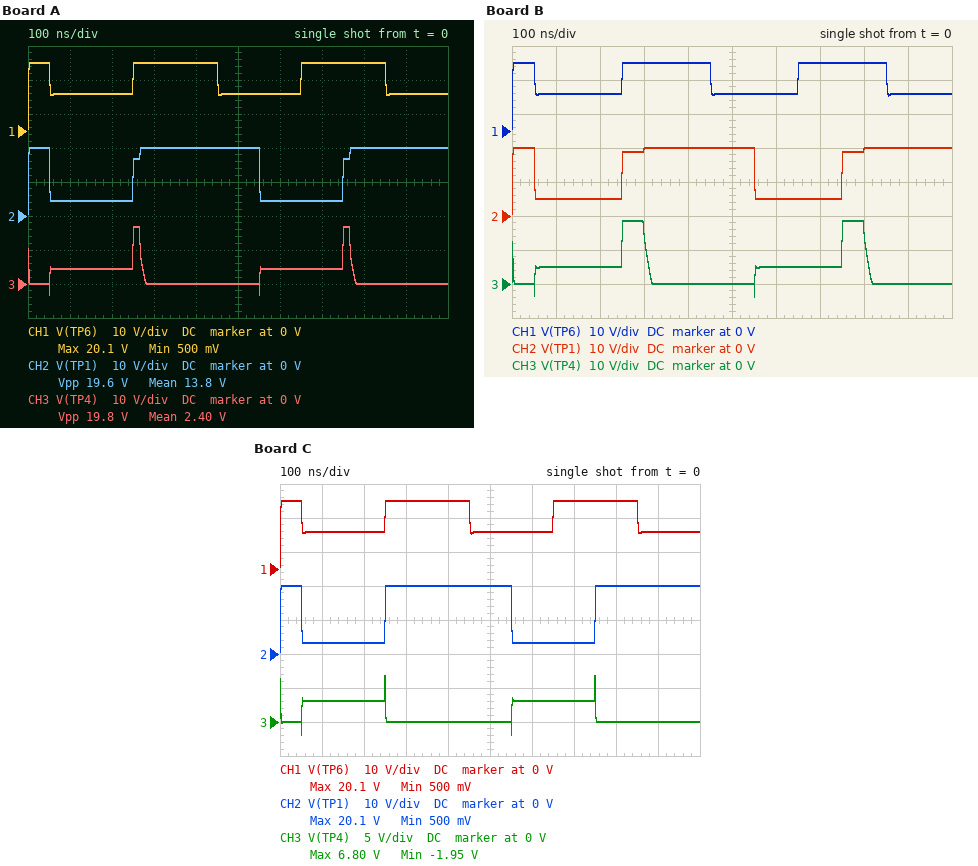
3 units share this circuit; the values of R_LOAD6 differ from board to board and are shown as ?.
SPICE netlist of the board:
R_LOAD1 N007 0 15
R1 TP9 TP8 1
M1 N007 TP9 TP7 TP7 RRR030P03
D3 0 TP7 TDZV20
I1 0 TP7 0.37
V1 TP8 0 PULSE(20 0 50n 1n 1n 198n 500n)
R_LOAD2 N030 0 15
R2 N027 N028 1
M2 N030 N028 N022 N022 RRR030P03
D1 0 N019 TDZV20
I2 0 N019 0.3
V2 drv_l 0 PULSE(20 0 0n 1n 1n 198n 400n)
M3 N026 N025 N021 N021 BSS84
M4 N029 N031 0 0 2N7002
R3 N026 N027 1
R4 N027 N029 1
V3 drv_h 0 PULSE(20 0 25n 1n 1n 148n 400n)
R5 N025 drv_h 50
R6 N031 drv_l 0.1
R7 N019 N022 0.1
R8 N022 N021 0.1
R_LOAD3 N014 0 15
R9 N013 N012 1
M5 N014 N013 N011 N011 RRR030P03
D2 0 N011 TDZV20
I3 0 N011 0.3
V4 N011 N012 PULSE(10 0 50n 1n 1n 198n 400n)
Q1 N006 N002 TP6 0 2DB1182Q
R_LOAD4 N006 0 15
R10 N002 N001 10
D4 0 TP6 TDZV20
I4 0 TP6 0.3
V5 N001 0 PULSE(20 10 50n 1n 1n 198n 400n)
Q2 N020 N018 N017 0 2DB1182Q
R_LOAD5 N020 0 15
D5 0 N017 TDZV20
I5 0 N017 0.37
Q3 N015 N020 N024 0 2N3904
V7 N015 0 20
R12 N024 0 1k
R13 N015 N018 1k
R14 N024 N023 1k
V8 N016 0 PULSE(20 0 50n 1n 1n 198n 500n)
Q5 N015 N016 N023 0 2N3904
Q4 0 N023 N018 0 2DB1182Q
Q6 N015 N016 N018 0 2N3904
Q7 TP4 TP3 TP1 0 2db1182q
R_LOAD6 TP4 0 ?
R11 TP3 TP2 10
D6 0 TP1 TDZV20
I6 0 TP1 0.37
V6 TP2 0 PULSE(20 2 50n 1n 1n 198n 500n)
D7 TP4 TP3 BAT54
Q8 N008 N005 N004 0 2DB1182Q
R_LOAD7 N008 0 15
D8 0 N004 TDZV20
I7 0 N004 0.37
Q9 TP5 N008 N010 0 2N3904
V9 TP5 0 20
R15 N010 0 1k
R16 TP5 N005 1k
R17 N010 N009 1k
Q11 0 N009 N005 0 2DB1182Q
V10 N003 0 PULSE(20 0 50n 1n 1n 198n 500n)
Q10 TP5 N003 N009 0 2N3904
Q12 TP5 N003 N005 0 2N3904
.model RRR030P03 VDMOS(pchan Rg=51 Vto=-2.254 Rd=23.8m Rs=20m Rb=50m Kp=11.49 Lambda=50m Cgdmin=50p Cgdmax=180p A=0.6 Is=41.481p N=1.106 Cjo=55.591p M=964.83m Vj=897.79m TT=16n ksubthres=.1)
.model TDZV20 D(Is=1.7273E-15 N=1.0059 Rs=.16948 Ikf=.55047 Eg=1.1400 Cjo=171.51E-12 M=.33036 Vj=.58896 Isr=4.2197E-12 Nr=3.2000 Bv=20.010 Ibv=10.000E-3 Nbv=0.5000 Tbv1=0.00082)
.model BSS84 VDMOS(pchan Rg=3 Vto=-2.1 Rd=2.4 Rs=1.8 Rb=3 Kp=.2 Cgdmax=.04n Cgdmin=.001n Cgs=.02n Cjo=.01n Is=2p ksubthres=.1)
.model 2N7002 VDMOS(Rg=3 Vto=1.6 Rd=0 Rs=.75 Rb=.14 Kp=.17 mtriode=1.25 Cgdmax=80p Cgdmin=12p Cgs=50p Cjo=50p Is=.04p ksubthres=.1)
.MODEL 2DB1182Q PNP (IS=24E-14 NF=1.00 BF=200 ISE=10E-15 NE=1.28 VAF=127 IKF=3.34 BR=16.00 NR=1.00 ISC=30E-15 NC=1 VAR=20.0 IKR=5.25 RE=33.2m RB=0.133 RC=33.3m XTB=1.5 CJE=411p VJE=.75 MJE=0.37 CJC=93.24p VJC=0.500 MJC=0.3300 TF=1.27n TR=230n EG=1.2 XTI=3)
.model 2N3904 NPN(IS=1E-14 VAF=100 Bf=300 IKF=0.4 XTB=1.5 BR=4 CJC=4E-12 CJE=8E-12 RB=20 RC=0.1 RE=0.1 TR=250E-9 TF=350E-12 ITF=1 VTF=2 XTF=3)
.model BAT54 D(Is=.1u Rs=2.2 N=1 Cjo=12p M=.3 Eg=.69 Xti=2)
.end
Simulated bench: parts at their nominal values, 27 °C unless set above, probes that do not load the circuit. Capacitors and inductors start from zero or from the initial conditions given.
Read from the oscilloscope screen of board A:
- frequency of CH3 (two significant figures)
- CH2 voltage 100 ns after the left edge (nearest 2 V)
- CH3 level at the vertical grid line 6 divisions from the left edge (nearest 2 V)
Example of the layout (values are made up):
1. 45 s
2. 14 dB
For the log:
1. 2.0 MHz
2. 4 V
3. 4 V
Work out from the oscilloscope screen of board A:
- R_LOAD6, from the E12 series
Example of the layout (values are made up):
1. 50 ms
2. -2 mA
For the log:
1. 22 Ω
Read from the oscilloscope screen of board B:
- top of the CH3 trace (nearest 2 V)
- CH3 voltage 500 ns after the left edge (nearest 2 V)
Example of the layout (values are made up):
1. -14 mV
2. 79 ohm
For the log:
1. 18 V
2. 0 V
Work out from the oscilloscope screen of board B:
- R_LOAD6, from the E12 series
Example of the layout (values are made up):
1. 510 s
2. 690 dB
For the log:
1. 33 Ω
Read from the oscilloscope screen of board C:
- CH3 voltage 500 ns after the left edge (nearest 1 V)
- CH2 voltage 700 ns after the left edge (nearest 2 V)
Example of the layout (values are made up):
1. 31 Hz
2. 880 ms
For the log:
1. 0 V
2. 4 V
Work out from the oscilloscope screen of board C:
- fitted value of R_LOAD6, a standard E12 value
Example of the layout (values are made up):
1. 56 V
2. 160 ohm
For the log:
1. 10 Ω
